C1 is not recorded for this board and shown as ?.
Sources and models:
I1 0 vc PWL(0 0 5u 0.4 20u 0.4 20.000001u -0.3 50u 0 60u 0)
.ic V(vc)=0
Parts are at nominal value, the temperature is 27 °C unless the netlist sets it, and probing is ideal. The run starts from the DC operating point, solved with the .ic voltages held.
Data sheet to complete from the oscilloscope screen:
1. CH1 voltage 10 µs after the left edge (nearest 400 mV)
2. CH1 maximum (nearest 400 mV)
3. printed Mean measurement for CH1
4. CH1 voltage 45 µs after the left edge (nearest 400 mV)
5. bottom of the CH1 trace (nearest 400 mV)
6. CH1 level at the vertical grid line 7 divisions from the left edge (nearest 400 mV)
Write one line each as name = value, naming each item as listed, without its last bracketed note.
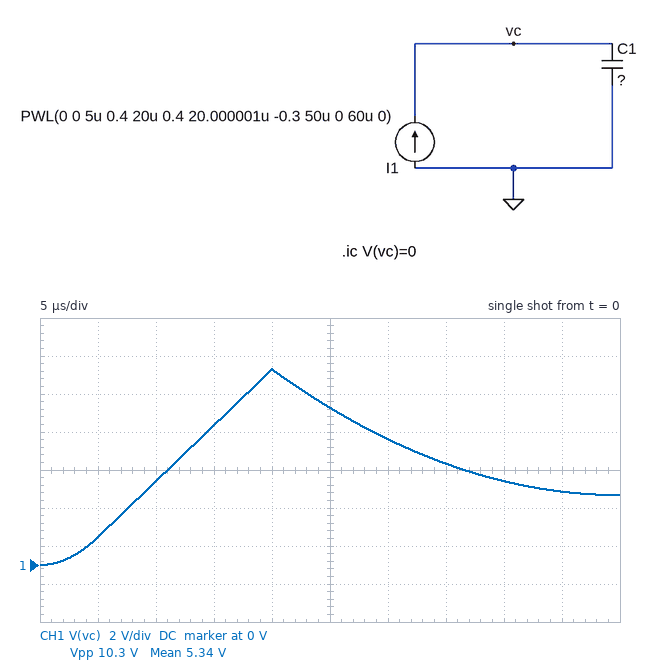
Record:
CH1 voltage 10 µs after the left edge = 4.4 V
CH1 maximum = 10.4 V
printed Mean measurement for CH1 = 5.34 V
CH1 voltage 45 µs after the left edge = 4.0 V
bottom of the CH1 trace = 0 V
CH1 level at the vertical grid line 7 divisions from the left edge = 5.2 V
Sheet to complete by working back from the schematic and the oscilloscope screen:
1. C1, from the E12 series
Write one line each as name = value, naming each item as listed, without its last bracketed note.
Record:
C1, from the E12 series = 680 nF
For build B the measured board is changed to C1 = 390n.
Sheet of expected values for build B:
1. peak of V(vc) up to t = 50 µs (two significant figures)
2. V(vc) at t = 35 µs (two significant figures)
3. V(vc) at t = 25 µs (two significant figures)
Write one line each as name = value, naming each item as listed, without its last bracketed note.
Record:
peak of V(vc) up to t = 50 µs = 18 V
V(vc) at t = 35 µs = 9.3 V
V(vc) at t = 25 µs = 14 V
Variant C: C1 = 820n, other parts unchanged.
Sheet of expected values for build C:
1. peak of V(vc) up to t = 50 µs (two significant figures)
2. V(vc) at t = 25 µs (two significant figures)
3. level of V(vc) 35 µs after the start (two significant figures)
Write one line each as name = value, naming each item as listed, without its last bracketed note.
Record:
peak of V(vc) up to t = 50 µs = 8.5 V
V(vc) at t = 25 µs = 6.9 V
level of V(vc) 35 µs after the start = 4.4 V
